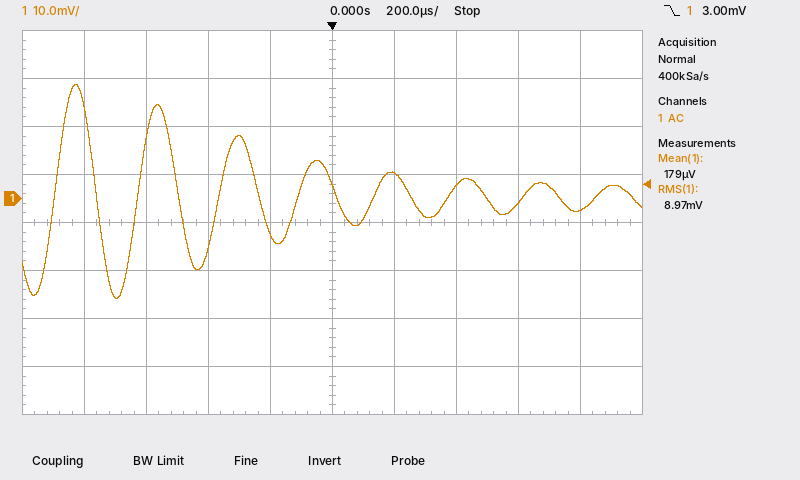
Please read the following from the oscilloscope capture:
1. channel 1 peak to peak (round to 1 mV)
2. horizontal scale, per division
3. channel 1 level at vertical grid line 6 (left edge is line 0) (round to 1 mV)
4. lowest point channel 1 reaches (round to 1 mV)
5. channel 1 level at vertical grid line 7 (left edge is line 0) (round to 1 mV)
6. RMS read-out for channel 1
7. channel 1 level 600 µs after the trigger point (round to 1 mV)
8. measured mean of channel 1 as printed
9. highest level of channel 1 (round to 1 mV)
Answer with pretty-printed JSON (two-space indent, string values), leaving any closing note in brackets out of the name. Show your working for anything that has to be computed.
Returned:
{
  "channel 1 peak to peak": "24 mV − (-21 mV) = 45 mV",
  "horizontal scale, per division": "200 µs",
  "channel 1 level at vertical grid line 6 (left edge is line 0)": "5 mV",
  "lowest point channel 1 reaches": "-21 mV",
  "channel 1 level at vertical grid line 7 (left edge is line 0)": "3 mV",
  "RMS read-out for channel 1": "8.97 mV",
  "channel 1 level 600 µs after the trigger point": "-1 mV",
  "measured mean of channel 1 as printed": "179 µV",
  "highest level of channel 1": "24 mV"
}
